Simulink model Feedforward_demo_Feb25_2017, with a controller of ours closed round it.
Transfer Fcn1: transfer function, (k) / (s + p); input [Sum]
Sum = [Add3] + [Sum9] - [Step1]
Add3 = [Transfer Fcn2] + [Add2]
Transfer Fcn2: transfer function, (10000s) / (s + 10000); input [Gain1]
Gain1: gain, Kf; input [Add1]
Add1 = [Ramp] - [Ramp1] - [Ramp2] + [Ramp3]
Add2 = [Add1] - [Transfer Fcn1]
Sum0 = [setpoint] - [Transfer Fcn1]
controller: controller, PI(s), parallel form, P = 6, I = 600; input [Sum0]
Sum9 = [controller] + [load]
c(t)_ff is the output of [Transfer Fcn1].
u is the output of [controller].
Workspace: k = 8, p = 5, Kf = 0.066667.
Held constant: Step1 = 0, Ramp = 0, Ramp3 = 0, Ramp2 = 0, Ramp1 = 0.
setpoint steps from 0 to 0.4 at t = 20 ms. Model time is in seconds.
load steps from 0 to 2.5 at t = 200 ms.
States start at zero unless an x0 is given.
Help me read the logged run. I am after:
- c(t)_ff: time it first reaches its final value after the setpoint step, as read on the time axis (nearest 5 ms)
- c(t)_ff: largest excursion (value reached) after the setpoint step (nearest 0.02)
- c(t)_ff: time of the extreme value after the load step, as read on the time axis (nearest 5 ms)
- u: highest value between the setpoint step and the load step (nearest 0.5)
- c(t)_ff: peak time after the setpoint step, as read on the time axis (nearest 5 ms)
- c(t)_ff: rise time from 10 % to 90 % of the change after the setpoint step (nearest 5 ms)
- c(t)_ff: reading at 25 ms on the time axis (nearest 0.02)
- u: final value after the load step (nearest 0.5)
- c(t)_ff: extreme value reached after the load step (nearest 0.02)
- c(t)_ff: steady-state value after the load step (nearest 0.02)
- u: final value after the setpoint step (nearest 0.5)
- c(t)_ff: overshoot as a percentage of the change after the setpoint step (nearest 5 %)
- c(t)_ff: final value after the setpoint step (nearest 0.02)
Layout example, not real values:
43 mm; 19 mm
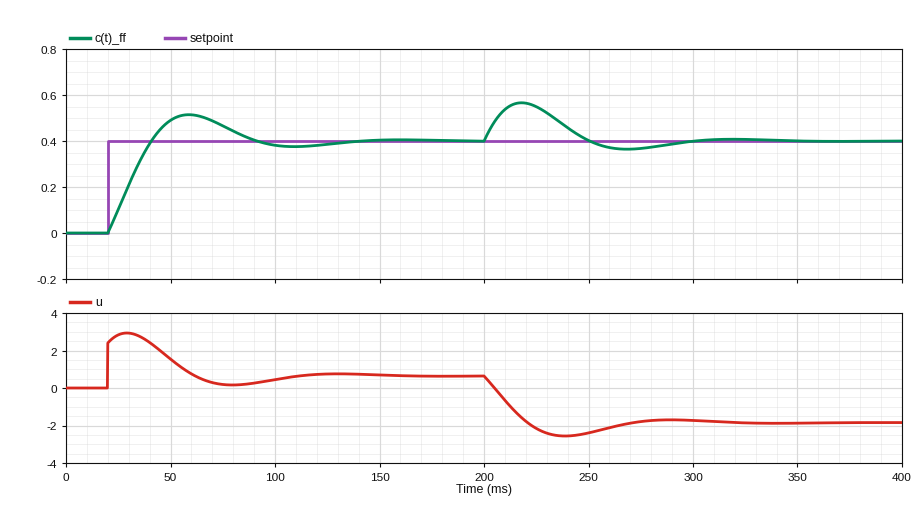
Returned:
40 ms; 0.52; 220 ms; 3.0; 60 ms; 15 ms; 0.10; -2.0; 0.56; 0.40; 0.5; 30 %; 0.40
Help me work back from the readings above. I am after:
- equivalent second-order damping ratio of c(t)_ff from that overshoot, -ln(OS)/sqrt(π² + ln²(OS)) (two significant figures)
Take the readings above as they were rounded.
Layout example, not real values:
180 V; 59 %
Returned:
0.36
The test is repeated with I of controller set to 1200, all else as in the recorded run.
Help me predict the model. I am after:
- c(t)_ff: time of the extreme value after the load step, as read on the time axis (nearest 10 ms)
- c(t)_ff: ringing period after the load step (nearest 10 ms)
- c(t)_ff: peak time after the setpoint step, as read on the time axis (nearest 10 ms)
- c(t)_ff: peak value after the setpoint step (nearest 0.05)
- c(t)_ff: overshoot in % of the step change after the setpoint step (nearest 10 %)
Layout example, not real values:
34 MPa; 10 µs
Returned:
210 ms; 70 ms; 50 ms; 0.55; 40 %
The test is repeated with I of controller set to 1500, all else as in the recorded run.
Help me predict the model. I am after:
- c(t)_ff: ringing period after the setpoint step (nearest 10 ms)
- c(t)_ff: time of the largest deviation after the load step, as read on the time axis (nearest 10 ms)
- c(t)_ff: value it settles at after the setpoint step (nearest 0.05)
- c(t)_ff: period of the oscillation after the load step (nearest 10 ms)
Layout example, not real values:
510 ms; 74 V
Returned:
60 ms; 210 ms; 0.40; 60 ms
